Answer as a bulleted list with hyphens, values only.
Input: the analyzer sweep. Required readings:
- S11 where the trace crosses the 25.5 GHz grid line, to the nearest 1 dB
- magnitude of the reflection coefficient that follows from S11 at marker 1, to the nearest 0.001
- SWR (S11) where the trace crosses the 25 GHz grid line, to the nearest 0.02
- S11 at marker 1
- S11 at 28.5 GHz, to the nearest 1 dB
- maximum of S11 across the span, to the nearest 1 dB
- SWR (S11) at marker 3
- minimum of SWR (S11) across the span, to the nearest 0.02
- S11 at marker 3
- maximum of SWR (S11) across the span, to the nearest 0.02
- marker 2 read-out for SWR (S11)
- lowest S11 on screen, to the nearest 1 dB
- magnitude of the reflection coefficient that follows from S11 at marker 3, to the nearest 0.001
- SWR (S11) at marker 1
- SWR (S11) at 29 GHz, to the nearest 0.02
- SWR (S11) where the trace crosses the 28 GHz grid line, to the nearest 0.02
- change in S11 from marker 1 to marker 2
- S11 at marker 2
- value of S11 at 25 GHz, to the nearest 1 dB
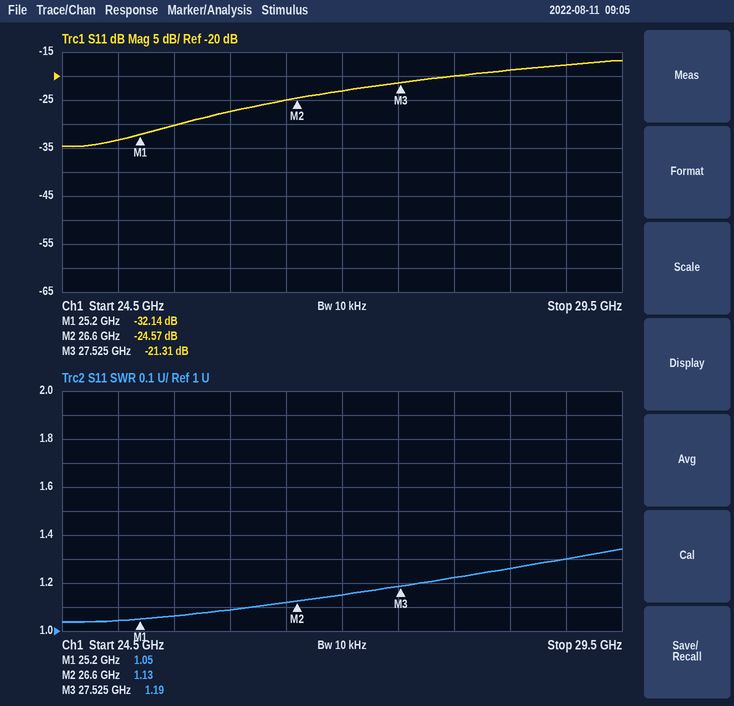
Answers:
- -30 dB
- 0.025
- 1.04
- -32.14 dB
- -19 dB
- -17 dB
- 1.19
- 1.04
- -21.31 dB
- 1.34
- 1.13
- -35 dB
- 0.086
- 1.05
- 1.30
- 1.22
- 7.57 dB
- -24.57 dB
- -33 dB
